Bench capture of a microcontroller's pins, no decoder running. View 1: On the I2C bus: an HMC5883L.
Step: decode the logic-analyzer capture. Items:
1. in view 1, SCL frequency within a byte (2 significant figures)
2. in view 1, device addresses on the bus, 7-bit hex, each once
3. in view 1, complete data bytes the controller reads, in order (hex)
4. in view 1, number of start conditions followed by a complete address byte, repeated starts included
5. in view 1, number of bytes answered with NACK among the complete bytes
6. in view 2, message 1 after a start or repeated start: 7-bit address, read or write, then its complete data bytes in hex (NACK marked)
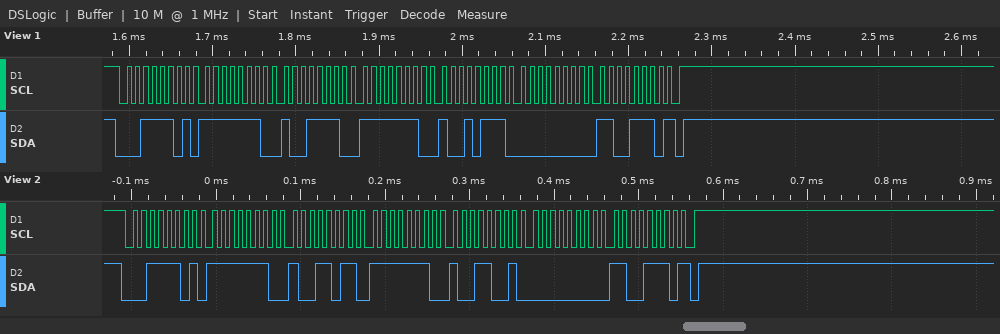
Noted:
100 kHz
0x1E
FE 9E FE 97 00 CE
1
1
0x1E read: FE 9B FE 99 00 CE NACK
